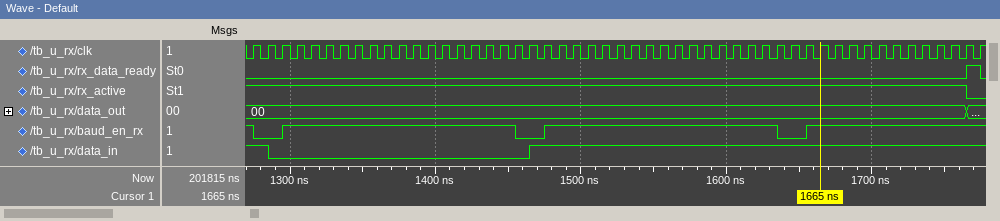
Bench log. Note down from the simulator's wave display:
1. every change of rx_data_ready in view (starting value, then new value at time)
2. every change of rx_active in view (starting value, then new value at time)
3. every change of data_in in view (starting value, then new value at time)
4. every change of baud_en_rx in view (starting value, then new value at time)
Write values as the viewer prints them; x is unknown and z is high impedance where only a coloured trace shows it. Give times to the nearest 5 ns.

0, 1 at 1765 ns, 0 at 1775 ns
1, 0 at 1765 ns
1, 0 at 1285 ns, 1 at 1465 ns
1, 0 at 1275 ns, 1 at 1295 ns, 0 at 1455 ns, 1 at 1475 ns, 0 at 1635 ns, 1 at 1655 ns
